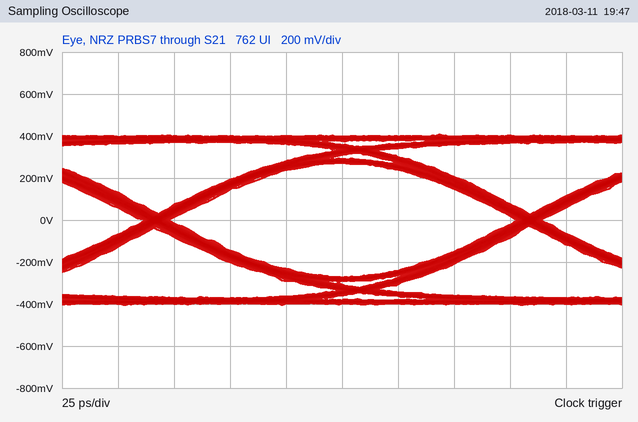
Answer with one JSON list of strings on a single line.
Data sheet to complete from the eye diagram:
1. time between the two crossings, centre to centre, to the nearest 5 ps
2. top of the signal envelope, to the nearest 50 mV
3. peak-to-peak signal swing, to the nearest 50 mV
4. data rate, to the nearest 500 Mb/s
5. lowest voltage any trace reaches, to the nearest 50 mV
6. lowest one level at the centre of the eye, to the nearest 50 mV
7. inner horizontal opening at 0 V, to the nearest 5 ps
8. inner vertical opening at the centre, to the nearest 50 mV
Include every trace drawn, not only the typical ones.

["165 ps", "400 mV", "800 mV", "6.0 Gb/s", "-400 mV", "250 mV", "155 ps", "550 mV"]
